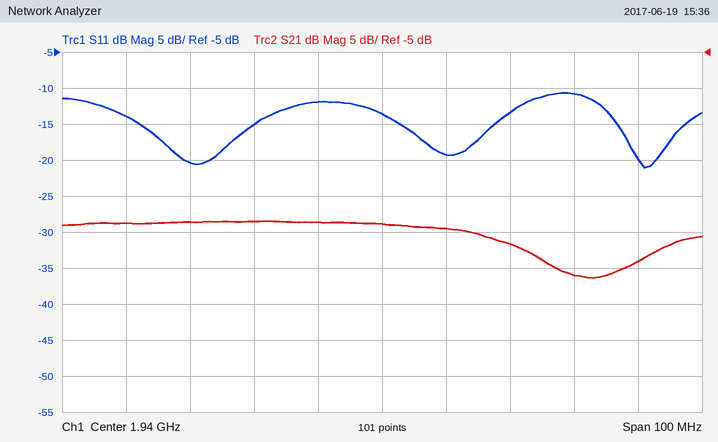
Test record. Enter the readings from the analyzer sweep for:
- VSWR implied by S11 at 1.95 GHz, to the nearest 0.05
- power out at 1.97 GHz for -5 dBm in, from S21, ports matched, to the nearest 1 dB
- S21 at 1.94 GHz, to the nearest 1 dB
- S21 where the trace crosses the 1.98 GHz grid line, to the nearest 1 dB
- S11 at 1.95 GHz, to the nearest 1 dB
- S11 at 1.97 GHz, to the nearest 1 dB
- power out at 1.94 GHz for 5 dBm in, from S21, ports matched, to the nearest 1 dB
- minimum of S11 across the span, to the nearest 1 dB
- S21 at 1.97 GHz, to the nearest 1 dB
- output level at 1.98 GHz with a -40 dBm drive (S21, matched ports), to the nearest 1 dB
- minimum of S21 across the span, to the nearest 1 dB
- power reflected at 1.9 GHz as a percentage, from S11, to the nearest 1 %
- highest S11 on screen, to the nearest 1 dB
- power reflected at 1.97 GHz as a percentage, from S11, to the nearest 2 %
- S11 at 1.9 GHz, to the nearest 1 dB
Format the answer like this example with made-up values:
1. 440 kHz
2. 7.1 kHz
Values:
1. 1.25
2. -41 dBm
3. -29 dB
4. -34 dB
5. -19 dB
6. -11 dB
7. -24 dBm
8. -21 dB
9. -36 dB
10. -74 dBm
11. -36 dB
12. 4 %
13. -11 dB
14. 8 %
15. -14 dB
